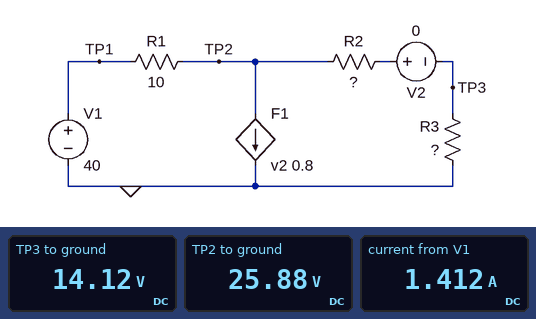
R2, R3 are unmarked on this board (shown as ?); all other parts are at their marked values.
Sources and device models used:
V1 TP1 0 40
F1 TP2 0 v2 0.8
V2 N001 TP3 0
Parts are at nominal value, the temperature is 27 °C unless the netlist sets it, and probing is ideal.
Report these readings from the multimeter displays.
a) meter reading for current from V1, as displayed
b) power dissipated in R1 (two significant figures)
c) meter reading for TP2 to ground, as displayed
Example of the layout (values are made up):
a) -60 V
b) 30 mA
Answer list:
a) 1.412 A
b) 20 W
c) 25.88 V
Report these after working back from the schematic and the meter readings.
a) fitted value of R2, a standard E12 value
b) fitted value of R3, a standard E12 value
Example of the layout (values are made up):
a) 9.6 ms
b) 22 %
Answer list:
a) 15 Ω
b) 18 Ω
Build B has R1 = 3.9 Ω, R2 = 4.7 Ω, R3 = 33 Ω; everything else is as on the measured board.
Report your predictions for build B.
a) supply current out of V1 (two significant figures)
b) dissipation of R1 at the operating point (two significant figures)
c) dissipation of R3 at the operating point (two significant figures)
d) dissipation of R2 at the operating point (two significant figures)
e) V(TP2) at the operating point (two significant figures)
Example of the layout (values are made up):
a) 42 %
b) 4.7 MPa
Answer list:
a) 1.6 A
b) 10 W
c) 26 W
d) 3.8 W
e) 34 V
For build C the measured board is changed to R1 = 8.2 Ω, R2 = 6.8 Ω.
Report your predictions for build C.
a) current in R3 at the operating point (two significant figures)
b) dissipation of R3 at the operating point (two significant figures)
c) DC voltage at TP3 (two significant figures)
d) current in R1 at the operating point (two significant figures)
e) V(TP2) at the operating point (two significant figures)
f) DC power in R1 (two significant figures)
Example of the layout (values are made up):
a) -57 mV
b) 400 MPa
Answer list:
a) 1.0 A
b) 18 W
c) 18 V
d) 1.8 A
e) 25 V
f) 27 W
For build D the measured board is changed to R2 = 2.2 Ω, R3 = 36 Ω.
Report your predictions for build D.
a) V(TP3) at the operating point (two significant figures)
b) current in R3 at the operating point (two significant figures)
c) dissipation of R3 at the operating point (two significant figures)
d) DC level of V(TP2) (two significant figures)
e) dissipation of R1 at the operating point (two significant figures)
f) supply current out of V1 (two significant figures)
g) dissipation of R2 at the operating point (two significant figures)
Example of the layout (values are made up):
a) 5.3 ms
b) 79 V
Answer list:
a) 26 V
b) 710 mA
c) 18 W
d) 27 V
e) 16 W
f) 1.3 A
g) 1.1 W
